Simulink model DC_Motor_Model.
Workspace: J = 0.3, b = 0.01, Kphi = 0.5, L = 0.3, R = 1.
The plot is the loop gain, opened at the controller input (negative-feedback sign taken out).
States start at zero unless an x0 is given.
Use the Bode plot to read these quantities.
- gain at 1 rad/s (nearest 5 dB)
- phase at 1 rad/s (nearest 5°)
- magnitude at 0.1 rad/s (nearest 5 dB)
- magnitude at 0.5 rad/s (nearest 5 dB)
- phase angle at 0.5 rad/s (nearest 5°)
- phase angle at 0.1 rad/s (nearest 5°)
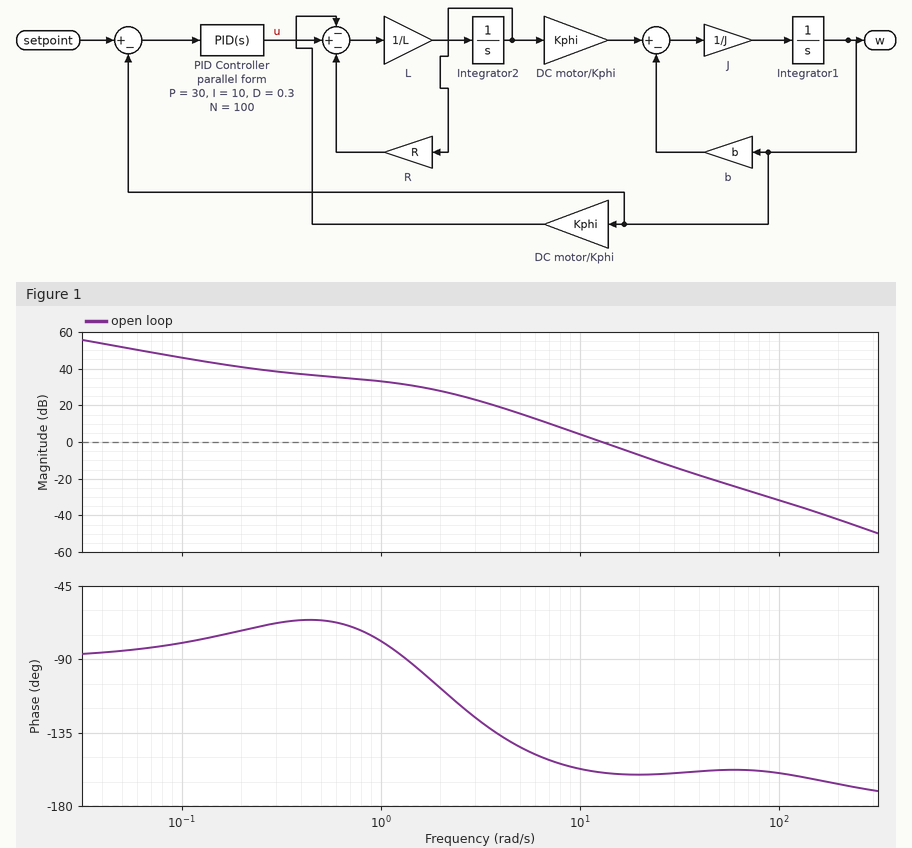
35 dB
-80°
45 dB
35 dB
-65°
-80°
